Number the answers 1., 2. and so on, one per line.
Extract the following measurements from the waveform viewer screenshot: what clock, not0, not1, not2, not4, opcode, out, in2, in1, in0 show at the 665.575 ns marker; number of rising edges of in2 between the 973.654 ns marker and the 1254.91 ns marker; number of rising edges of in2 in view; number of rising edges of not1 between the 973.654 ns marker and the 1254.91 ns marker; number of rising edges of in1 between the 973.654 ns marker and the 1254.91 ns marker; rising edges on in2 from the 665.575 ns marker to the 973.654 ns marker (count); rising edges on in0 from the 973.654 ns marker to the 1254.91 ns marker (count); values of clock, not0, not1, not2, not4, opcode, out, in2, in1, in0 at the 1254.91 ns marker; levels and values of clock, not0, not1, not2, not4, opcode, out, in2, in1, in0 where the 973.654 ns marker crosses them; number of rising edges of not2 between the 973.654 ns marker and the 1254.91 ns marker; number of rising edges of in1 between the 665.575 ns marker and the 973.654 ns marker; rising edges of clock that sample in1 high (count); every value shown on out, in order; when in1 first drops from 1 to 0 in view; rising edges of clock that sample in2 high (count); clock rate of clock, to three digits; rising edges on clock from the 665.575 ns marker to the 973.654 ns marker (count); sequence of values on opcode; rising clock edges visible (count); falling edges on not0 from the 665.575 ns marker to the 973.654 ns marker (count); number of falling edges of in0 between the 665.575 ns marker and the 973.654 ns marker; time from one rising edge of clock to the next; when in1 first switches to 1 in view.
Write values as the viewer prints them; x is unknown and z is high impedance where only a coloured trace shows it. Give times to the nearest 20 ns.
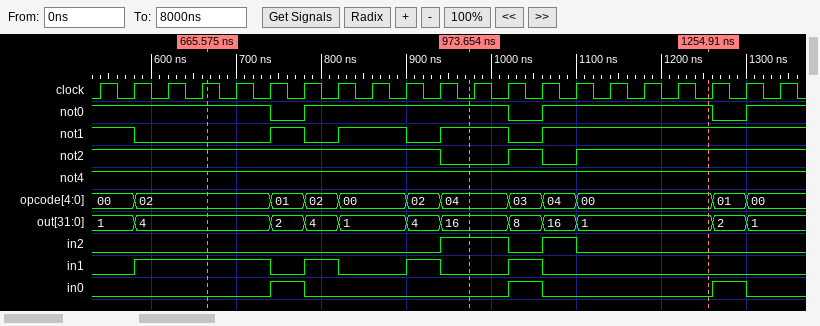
1. clock=1, not0=1, not1=0, not2=1, not4=1, opcode=02, out=4, in2=0, in1=1, in0=0
2. 1
3. 2
4. 1
5. 1
6. 1
7. 1
8. clock=0, not0=1, not1=1, not2=1, not4=1, opcode=00, out=1, in2=0, in1=0, in0=0
9. clock=0, not0=1, not1=1, not2=0, not4=1, opcode=04, out=16, in2=1, in1=0, in0=0
10. 2
11. 2
12. 7
13. 1, 4, 2, 4, 1, 4, 16, 8, 16, 1, 2, 1
14. 740 ns
15. 3
16. 25.0 MHz
17. 7
18. 00, 02, 01, 02, 00, 02, 04, 03, 04, 00, 01, 00
19. 21
20. 1
21. 1
22. 40 ns
23. 580 ns
